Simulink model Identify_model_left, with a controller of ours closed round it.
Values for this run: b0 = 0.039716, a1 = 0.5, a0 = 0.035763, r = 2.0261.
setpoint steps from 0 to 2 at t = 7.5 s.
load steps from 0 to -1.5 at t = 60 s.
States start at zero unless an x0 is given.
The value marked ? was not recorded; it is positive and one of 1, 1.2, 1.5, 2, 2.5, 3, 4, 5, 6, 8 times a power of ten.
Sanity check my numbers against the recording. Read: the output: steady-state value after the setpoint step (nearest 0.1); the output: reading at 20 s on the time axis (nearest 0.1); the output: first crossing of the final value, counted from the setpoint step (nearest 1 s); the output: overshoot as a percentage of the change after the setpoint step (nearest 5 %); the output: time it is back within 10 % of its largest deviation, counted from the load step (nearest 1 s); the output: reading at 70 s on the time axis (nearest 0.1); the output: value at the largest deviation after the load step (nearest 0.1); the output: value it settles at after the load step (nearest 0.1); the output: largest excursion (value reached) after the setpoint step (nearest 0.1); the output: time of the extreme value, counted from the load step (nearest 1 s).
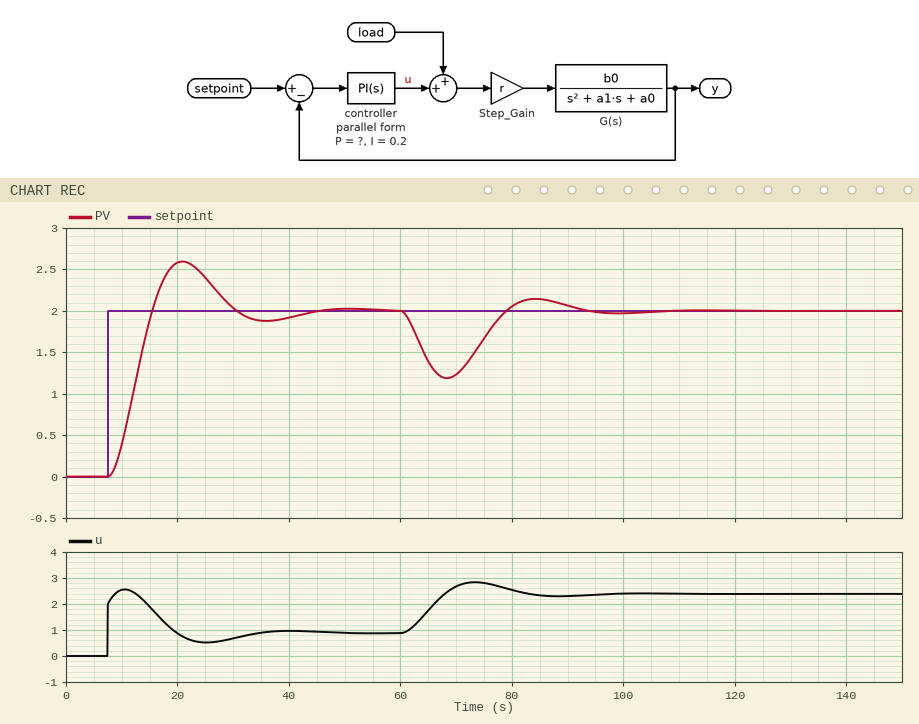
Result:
2.0
2.6
8 s
30 %
29 s
1.2
1.2
2.0
2.6
8 s
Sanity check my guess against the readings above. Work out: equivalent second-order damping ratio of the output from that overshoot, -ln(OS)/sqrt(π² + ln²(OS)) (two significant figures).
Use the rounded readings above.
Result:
0.36
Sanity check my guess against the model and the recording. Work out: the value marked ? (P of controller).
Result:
1
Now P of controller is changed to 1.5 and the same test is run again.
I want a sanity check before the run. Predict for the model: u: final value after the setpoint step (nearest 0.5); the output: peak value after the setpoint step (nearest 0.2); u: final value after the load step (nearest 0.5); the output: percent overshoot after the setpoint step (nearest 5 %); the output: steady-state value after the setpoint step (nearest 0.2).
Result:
1.0
2.4
2.5
20 %
2.0
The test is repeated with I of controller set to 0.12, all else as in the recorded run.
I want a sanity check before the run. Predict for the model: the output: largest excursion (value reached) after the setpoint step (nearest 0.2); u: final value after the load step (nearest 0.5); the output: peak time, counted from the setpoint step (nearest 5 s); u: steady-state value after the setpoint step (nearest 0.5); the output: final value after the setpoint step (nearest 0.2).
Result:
2.2
2.5
15 s
1.0
2.0
